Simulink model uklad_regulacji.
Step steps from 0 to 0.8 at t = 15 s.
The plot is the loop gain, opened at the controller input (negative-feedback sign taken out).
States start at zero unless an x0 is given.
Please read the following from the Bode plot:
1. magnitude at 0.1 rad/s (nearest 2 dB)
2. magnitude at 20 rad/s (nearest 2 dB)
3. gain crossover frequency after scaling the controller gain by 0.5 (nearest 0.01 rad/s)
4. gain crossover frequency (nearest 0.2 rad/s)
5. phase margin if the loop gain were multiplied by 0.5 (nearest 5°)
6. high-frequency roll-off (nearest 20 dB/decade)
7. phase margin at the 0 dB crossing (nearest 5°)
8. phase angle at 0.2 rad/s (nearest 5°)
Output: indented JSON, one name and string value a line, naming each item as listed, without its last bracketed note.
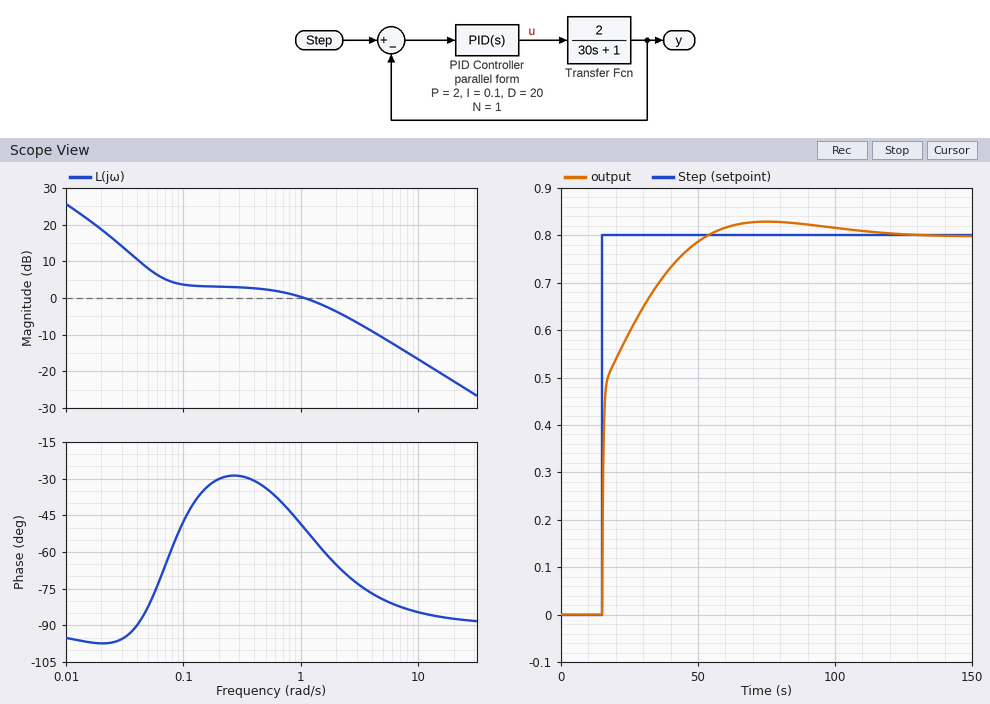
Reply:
{
  "magnitude at 0.1 rad/s": "4 dB",
  "magnitude at 20 rad/s": "-22 dB",
  "gain crossover frequency after scaling the controller gain by 0.5": "0.06 rad/s",
  "gain crossover frequency": "1.0 rad/s",
  "phase margin if the loop gain were multiplied by 0.5": "110°",
  "high-frequency roll-off": "-20 dB/decade",
  "phase margin at the 0 dB crossing": "130°",
  "phase angle at 0.2 rad/s": "-30°"
}
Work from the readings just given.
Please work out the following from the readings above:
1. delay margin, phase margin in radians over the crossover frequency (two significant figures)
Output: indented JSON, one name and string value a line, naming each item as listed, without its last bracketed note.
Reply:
{
  "delay margin, phase margin in radians over the crossover frequency": "2.3 s"
}
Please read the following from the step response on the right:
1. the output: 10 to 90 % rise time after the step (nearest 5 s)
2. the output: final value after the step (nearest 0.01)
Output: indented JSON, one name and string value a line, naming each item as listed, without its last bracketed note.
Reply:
{
  "the output: 10 to 90 % rise time after the step": "25 s",
  "the output: final value after the step": "0.80"
}
